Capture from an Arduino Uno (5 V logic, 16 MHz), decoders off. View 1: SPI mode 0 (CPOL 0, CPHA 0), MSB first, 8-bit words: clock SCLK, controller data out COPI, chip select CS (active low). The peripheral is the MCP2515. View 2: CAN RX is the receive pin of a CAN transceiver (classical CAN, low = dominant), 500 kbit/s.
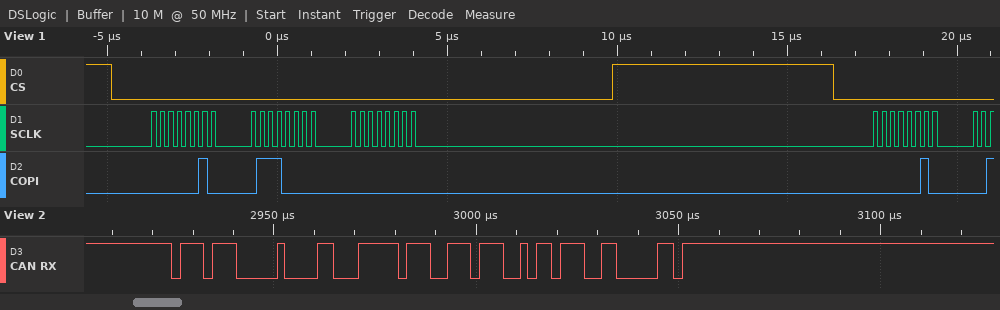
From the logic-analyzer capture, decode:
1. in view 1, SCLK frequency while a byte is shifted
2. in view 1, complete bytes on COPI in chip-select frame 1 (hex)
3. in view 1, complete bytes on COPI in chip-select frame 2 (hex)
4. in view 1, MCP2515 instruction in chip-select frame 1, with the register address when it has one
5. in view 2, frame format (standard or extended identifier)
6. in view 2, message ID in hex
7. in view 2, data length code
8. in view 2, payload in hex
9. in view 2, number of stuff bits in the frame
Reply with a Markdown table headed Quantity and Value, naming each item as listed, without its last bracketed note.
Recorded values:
| Quantity | Value |
|---|---|
| in view 1, SCLK frequency while a byte is shifted | 4 MHz |
| in view 1, complete bytes on COPI in chip-select frame 1 | 0x02 0x70 0x00 |
| in view 1, complete bytes on COPI in chip-select frame 2 | 0x02 |
| in view 1, MCP2515 instruction in chip-select frame 1, with the register address when it has one | WRITE 0x70 |
| in view 2, frame format | standard |
| in view 2, message ID in hex | 0x770 |
| in view 2, data length code | 3 |
| in view 2, payload in hex | 1F E7 72 |
| in view 2, number of stuff bits in the frame | 3 |
